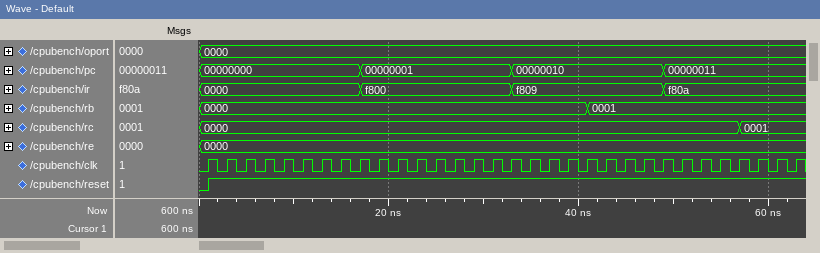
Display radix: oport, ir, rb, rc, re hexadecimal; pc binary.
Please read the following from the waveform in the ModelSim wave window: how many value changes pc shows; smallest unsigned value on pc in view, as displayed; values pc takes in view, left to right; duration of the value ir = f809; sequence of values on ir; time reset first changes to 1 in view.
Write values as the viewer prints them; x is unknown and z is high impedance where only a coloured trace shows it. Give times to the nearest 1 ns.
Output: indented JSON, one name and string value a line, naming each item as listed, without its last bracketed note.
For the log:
{
  "how many value changes pc shows": "3",
  "smallest unsigned value on pc in view, as displayed": "00000000",
  "values pc takes in view, left to right": "00000000, 00000001, 00000010, 00000011",
  "duration of the value ir = f809": "16 ns",
  "sequence of values on ir": "0000, f800, f809, f80a",
  "time reset first changes to 1 in view": "1 ns"
}
